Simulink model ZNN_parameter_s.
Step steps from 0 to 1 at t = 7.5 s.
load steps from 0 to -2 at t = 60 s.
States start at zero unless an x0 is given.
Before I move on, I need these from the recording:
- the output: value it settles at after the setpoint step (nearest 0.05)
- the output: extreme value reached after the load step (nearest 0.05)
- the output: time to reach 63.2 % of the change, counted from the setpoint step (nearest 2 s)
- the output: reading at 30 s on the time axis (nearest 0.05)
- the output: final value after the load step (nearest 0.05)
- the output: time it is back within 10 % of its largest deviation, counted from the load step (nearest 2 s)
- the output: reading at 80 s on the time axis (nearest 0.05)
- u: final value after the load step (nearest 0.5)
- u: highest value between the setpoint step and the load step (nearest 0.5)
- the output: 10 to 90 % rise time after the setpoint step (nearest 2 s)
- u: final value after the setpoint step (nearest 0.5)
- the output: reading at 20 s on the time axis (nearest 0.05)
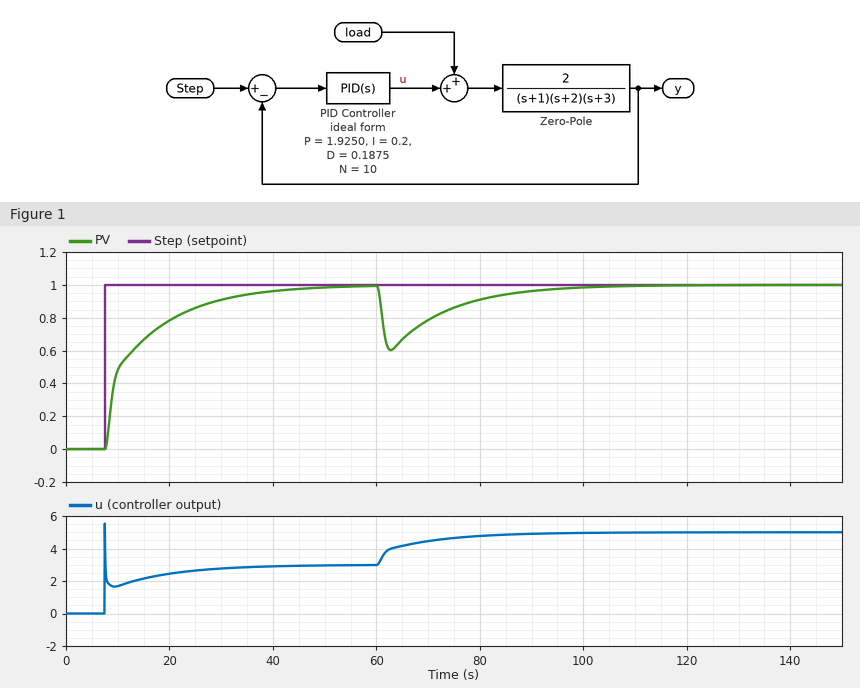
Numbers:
1.00
0.60
6 s
0.90
1.00
30 s
0.90
5.0
5.5
20 s
3.0
0.80
